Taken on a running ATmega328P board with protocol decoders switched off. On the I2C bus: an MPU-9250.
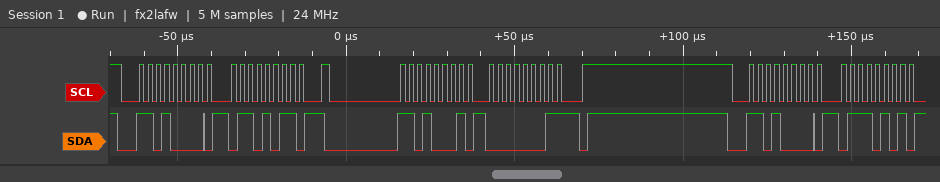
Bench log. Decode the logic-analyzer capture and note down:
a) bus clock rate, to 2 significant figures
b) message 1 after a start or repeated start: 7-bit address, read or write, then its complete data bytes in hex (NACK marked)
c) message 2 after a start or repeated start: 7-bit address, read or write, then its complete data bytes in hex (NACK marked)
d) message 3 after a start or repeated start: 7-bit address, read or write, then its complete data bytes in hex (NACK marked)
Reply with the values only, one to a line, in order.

400 kHz
0x68 write: 6B
0x68 read: 01 NACK
0x68 write: 75
